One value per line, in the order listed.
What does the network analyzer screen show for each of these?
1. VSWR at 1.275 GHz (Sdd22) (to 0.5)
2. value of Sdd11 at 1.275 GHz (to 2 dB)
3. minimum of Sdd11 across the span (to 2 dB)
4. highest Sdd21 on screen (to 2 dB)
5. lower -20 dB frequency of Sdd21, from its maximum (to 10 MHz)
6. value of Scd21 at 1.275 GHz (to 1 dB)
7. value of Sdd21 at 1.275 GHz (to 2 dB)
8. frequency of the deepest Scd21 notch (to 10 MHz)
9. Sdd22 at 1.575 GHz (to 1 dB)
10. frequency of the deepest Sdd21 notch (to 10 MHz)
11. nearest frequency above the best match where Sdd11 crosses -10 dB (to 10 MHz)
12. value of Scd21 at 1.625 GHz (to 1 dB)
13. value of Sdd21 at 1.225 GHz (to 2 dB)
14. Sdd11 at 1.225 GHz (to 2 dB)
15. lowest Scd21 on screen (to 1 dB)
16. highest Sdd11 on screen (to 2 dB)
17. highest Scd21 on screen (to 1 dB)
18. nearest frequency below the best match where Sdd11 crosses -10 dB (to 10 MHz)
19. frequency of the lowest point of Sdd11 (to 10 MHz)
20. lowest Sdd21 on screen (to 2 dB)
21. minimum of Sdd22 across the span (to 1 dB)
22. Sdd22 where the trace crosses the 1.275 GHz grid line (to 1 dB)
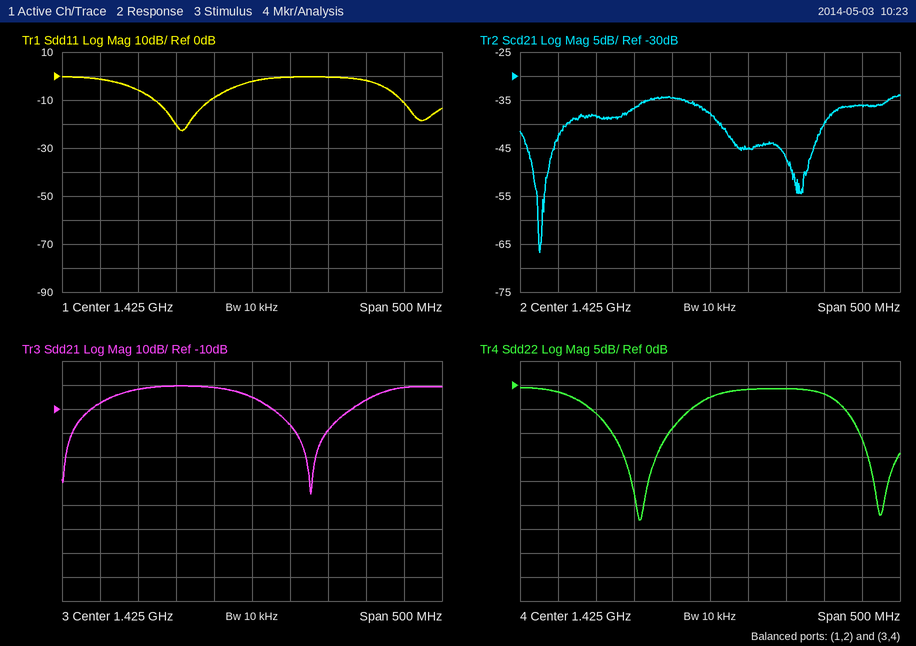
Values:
3.0
-6 dB
-22 dB
0 dB
1.19 GHz
-38 dB
-2 dB
1.20 GHz
-2 dB
1.50 GHz
1.37 GHz
-36 dB
-8 dB
-2 dB
-67 dB
0 dB
-34 dB
1.30 GHz
1.33 GHz
-46 dB
-28 dB
-6 dB
